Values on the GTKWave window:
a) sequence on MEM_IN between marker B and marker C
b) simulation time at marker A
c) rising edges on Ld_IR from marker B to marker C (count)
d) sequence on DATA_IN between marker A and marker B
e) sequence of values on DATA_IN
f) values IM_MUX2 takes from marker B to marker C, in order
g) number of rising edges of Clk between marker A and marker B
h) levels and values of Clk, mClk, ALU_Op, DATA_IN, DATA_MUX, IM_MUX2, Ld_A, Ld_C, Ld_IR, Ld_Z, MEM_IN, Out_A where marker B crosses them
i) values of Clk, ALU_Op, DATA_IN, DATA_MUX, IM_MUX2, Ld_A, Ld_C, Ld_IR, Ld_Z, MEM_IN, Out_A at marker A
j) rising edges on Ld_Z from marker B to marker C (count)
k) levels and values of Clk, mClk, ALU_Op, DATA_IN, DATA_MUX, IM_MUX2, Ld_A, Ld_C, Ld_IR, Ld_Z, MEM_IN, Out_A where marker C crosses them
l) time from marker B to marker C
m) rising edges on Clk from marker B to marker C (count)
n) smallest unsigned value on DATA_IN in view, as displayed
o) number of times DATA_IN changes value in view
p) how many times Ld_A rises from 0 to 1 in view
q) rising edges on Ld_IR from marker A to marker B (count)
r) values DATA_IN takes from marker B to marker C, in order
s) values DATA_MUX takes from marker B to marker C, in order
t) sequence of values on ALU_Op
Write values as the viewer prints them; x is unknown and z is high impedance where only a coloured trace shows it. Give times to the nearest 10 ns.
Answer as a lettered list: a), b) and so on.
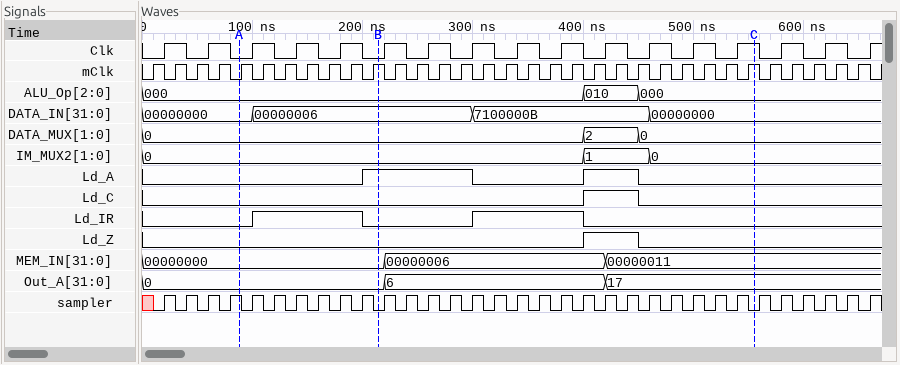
a) 00000000, 00000006, 00000011
b) 90 ns
c) 1
d) 00000000, 00000006
e) 00000000, 00000006, 7100000B, 00000000
f) 0, 1, 0
g) 3
h) Clk=0, mClk=1, ALU_Op=000, DATA_IN=00000006, DATA_MUX=0, IM_MUX2=0, Ld_A=1, Ld_C=0, Ld_IR=0, Ld_Z=0, MEM_IN=00000000, Out_A=0
i) Clk=0, ALU_Op=000, DATA_IN=00000000, DATA_MUX=0, IM_MUX2=0, Ld_A=0, Ld_C=0, Ld_IR=0, Ld_Z=0, MEM_IN=00000000, Out_A=0
j) 1
k) Clk=1, mClk=1, ALU_Op=000, DATA_IN=00000000, DATA_MUX=0, IM_MUX2=0, Ld_A=0, Ld_C=0, Ld_IR=0, Ld_Z=0, MEM_IN=00000011, Out_A=17
l) 340 ns
m) 9
n) 00000000
o) 3
p) 2
q) 1
r) 00000006, 7100000B, 00000000
s) 0, 2, 0
t) 000, 010, 000
